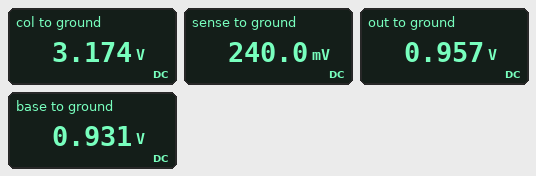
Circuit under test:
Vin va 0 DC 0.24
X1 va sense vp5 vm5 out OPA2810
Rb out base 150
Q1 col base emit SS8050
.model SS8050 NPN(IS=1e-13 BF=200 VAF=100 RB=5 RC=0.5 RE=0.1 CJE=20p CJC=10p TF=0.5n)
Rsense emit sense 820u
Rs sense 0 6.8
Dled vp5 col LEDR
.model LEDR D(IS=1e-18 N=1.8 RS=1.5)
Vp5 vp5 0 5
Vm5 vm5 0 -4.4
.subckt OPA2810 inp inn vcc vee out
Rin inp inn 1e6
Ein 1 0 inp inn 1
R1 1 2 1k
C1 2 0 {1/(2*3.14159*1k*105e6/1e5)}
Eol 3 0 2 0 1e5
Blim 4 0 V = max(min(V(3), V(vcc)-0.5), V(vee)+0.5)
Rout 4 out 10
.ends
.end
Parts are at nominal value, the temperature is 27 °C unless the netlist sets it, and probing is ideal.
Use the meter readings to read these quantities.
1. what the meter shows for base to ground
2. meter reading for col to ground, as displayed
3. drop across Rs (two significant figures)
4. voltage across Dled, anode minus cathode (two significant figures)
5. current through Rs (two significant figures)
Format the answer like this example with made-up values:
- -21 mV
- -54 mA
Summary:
- 0.931 V
- 3.174 V
- 240 mV
- 1.8 V
- 35 mA
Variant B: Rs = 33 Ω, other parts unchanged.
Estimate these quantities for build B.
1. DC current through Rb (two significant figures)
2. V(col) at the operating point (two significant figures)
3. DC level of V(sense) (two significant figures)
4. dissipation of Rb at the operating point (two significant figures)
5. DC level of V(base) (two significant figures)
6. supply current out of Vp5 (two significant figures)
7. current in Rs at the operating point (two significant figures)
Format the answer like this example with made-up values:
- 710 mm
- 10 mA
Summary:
- 35 µA
- 3.3 V
- 240 mV
- 190 nW
- 890 mV
- 7.2 mA
- 7.3 mA
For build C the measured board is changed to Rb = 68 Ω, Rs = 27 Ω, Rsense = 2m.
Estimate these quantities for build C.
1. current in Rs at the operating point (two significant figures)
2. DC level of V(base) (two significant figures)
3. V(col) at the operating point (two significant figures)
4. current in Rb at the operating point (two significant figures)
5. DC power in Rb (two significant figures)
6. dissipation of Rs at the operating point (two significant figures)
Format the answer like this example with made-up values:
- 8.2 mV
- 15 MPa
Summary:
- 8.9 mA
- 890 mV
- 3.3 V
- 43 µA
- 130 nW
- 2.1 mW
